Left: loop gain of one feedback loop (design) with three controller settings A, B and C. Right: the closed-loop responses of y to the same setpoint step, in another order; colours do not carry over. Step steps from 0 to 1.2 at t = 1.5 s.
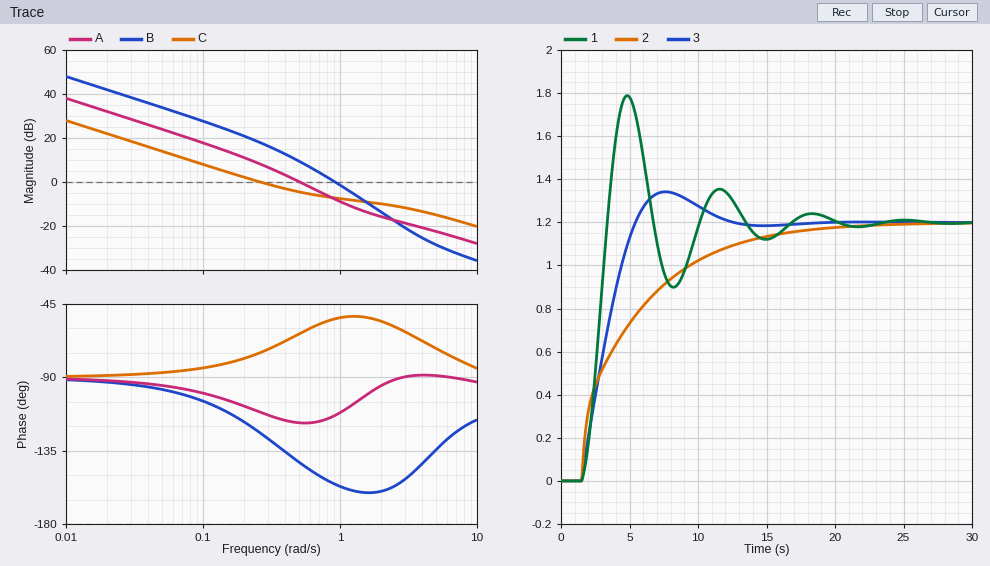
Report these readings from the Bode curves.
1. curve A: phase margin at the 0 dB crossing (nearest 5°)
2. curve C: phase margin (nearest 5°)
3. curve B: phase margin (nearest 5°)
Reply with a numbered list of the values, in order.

1. 60°
2. 105°
3. 25°
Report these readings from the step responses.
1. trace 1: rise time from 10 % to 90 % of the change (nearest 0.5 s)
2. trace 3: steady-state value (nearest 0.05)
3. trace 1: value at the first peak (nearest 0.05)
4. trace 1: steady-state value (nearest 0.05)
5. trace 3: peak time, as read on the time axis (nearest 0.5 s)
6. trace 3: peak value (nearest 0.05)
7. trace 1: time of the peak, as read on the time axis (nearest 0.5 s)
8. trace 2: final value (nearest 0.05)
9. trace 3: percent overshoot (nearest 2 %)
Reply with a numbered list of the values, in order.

1. 1.5 s
2. 1.20
3. 1.80
4. 1.20
5. 7.5 s
6. 1.35
7. 5.0 s
8. 1.20
9. 12 %
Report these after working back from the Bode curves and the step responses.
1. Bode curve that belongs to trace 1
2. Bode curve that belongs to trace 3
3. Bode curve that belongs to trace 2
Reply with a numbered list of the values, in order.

1. B
2. A
3. C
